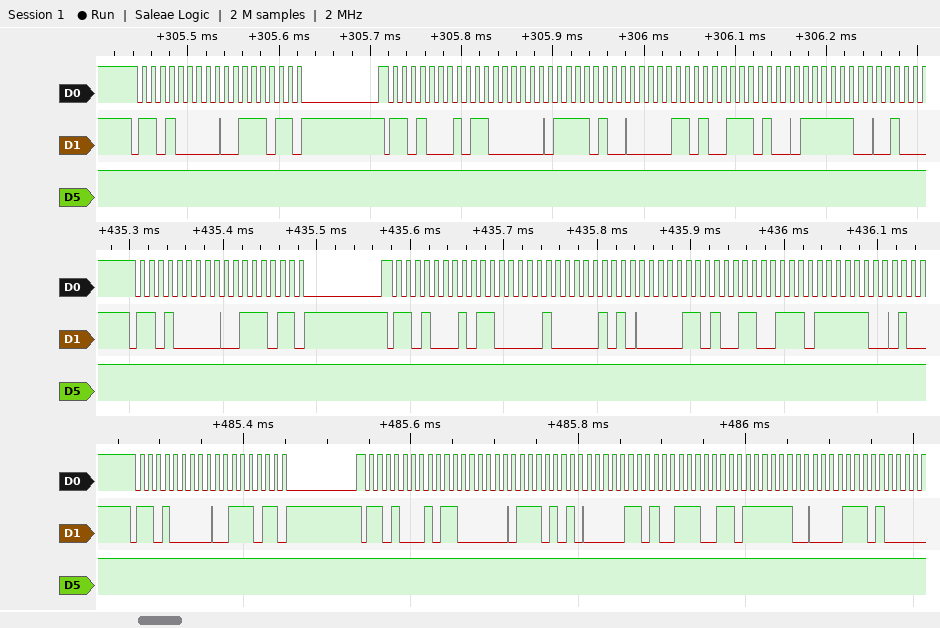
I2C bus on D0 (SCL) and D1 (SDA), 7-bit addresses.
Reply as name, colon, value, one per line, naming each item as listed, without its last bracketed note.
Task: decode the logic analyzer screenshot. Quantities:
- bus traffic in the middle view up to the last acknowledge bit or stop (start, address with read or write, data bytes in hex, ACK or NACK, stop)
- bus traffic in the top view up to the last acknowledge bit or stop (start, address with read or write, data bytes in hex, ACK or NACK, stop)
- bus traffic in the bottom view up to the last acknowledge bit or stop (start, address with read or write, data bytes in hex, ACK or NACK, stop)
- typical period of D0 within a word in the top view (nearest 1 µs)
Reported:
bus traffic in the middle view up to the last acknowledge bit or stop: start, address 68 write ACK, 3B ACK, repeated start, address 68 read ACK, C1 ACK, 0A ACK, 0D ACK, 67 ACK, FC ACK
bus traffic in the top view up to the last acknowledge bit or stop: start, address 68 write ACK, 3B ACK, repeated start, address 68 read ACK, C0 ACK, F4 ACK, 0D ACK, 74 ACK, FC ACK
bus traffic in the bottom view up to the last acknowledge bit or stop: start, address 68 write ACK, 3B ACK, repeated start, address 68 read ACK, C0 ACK, EA ACK, 0D ACK, 73 ACK, FC ACK, 1D ACK
typical period of D0 within a word in the top view: 10 µs
